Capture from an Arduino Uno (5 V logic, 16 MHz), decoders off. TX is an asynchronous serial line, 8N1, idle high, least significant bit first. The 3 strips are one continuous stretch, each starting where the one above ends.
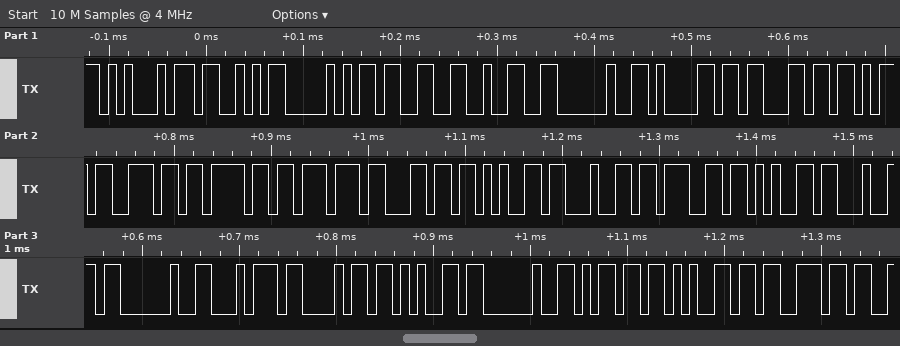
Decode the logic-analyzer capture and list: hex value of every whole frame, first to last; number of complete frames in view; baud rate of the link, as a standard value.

45 53 50 33 32 20 61 63 6B 6E 6F 77 6C 65 64 67 65 64 20 74 68 65 20 6D 65 73
26
115200 baud
